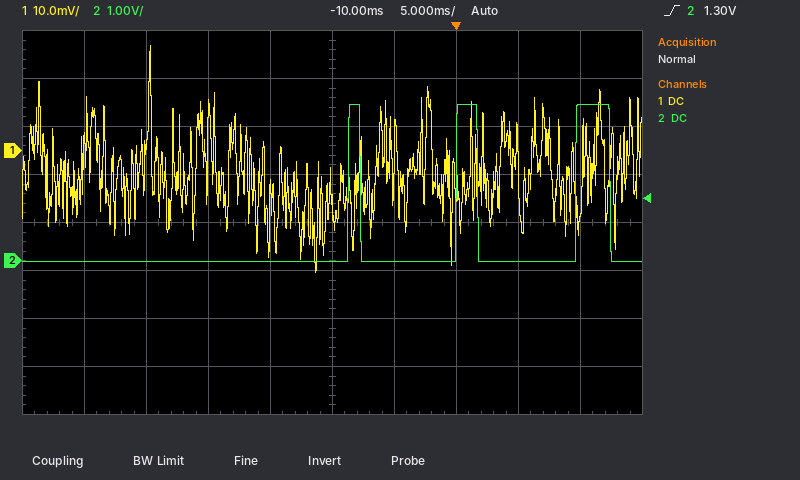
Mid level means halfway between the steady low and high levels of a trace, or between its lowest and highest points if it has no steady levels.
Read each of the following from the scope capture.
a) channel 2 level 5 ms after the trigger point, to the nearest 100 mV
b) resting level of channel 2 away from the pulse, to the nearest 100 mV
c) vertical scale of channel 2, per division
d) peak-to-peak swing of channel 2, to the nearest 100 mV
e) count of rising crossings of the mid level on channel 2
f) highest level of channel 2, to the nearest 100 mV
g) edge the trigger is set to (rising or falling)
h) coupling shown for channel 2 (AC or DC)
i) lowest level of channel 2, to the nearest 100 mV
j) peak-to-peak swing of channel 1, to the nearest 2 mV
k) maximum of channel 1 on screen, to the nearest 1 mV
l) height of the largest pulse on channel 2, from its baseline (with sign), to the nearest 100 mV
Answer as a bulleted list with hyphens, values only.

- 0.0 V
- 0.0 V
- 1 V
- 3.3 V
- 3
- 3.3 V
- rising
- DC
- 0.0 V
- 48 mV
- 22 mV
- +3.3 V
